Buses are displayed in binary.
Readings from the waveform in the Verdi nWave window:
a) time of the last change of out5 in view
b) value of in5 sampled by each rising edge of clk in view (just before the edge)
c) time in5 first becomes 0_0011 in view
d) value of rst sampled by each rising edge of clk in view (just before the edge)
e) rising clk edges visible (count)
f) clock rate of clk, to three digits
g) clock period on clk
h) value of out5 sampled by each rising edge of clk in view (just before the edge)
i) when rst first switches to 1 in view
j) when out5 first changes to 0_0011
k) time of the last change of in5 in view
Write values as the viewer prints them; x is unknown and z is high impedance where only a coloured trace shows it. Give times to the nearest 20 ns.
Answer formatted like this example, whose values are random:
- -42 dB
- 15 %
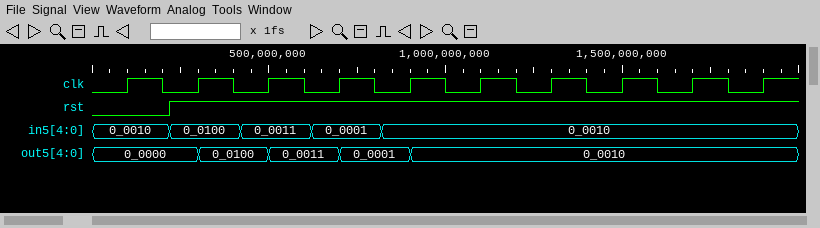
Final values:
- 900 ns
- 0_0010, 0_0100, 0_0011, 0_0001, 0_0010, 0_0010, 0_0010, 0_0010, 0_0010, 0_0010
- 420 ns
- 0 1 1 1 1 1 1 1 1 1
- 10
- 5.00 MHz
- 200 ns
- 0_0000, 0_0000, 0_0100, 0_0011, 0_0001, 0_0010, 0_0010, 0_0010, 0_0010, 0_0010
- 220 ns
- 500 ns
- 820 ns
